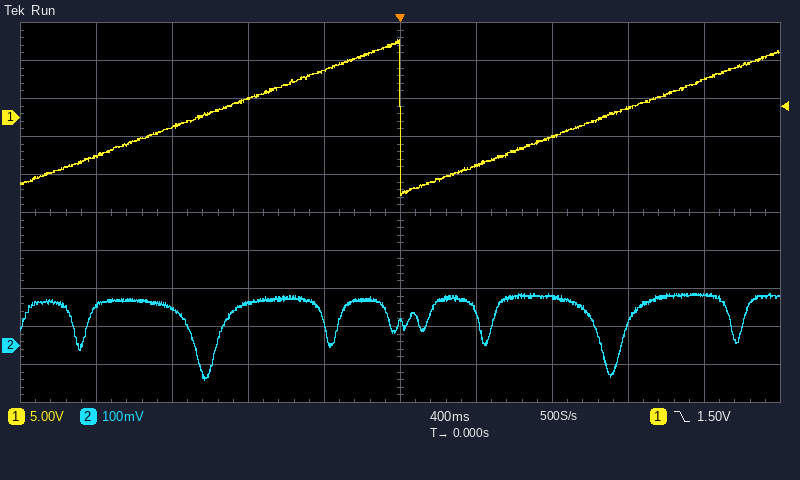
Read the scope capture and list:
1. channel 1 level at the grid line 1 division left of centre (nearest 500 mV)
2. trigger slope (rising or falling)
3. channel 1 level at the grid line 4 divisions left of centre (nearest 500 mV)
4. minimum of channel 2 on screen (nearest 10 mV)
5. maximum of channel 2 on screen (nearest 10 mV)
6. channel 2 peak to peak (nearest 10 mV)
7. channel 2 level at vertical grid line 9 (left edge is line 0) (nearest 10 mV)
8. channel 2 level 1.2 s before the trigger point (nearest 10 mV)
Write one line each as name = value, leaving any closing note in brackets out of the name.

channel 1 level at the grid line 1 division left of centre = 6.0 V
trigger slope = falling
channel 1 level at the grid line 4 divisions left of centre = -5.0 V
minimum of channel 2 on screen = -90 mV
maximum of channel 2 on screen = 140 mV
channel 2 peak to peak = 230 mV
channel 2 level at vertical grid line 9 (left edge is line 0) = 130 mV
channel 2 level 1.2 s before the trigger point = 100 mV
